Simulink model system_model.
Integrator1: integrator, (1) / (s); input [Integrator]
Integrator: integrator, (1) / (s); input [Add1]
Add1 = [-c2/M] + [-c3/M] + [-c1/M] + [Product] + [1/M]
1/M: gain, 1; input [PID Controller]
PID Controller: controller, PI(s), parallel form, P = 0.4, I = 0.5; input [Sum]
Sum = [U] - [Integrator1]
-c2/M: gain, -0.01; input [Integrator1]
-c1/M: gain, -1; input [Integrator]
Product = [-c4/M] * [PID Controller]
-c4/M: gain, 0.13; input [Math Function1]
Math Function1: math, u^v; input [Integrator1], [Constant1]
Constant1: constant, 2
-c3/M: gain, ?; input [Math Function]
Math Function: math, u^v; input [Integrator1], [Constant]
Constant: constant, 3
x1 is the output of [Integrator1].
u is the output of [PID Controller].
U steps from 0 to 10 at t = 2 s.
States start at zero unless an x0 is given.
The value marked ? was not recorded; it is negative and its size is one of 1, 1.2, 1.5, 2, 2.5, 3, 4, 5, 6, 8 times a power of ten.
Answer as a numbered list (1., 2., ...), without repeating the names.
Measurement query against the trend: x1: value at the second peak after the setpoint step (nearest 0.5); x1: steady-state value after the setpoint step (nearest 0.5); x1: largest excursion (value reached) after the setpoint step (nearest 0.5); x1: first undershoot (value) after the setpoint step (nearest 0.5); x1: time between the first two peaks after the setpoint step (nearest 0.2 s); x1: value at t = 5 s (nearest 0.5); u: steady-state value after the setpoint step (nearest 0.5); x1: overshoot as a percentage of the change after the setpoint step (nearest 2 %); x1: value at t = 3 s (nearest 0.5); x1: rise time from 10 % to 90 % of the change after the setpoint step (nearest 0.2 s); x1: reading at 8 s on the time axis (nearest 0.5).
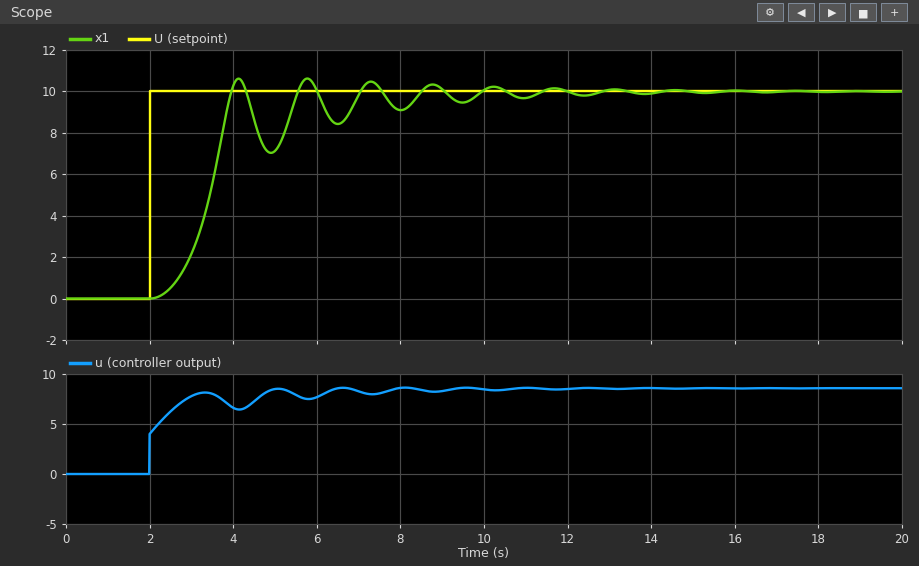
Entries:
1. 10.5
2. 10.0
3. 10.5
4. 7.0
5. 1.6 s
6. 7.0
7. 8.5
8. 6 %
9. 2.0
10. 1.2 s
11. 9.0
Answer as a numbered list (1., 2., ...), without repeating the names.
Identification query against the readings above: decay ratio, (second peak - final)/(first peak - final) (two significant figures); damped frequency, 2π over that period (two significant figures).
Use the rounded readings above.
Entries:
1. 1.0
2. 3.9 rad/s
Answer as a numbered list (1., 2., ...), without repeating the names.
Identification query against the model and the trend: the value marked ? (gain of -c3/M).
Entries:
1. -0.12
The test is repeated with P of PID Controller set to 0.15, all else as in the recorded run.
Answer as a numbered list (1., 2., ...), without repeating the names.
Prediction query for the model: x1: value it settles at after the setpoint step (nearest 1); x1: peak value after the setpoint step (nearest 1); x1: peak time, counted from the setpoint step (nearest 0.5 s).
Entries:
1. 10
2. 12
3. 2.5 s
